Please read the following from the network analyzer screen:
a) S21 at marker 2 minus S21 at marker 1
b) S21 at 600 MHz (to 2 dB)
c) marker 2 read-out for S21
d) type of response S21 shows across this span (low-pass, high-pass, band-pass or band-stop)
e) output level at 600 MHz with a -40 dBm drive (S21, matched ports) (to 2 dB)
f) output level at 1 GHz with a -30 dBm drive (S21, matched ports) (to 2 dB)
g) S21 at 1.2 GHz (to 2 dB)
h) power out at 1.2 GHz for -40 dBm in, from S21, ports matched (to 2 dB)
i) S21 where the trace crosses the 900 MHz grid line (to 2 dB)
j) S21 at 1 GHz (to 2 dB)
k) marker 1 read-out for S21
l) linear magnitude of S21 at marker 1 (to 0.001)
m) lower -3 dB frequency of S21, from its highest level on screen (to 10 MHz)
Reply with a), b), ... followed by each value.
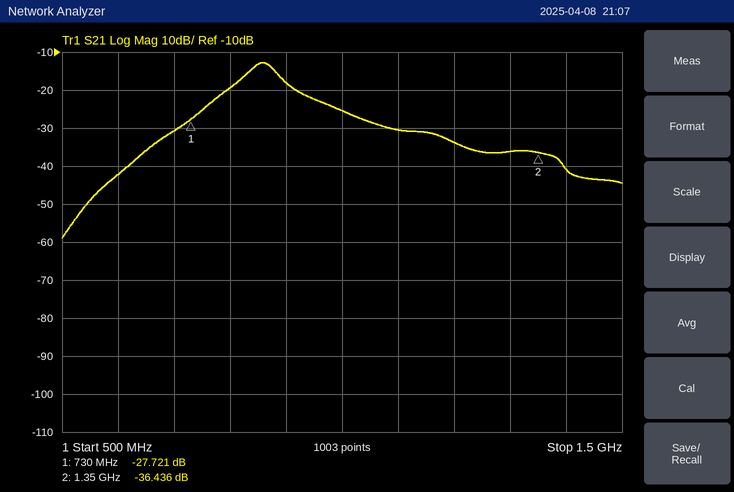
a) -8.715 dB
b) -42 dB
c) -36.436 dB
d) band-pass
e) -82 dBm
f) -56 dBm
g) -34 dB
h) -74 dBm
i) -18 dB
j) -26 dB
k) -27.721 dB
l) 0.041
m) 830 MHz
